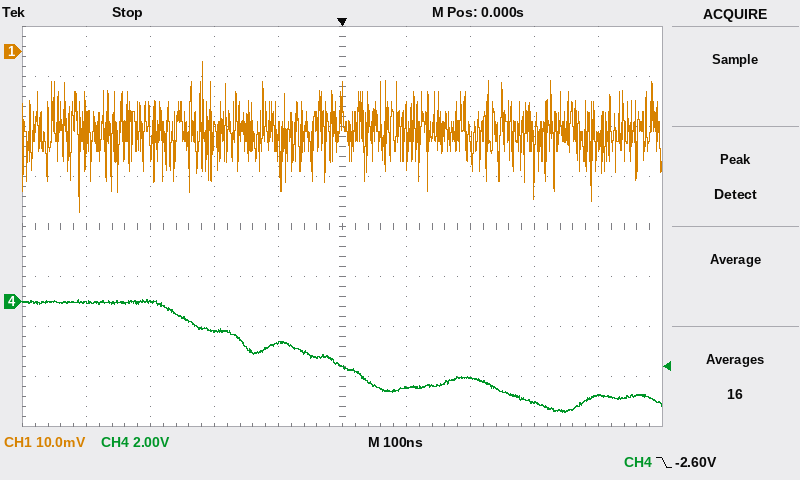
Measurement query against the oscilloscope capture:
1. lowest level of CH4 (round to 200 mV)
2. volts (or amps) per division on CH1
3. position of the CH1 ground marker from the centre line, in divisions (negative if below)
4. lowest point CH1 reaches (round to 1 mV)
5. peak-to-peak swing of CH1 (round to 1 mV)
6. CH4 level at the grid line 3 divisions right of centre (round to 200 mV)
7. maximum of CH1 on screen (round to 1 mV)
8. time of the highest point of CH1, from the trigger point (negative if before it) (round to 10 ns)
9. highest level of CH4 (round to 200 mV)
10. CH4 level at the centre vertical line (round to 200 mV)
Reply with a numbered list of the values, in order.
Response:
1. -4.4 V
2. 10 mV
3. +3.5 div
4. -32 mV
5. 30 mV
6. -4.0 V
7. -2 mV
8. -220 ns
9. 0.0 V
10. -2.6 V
